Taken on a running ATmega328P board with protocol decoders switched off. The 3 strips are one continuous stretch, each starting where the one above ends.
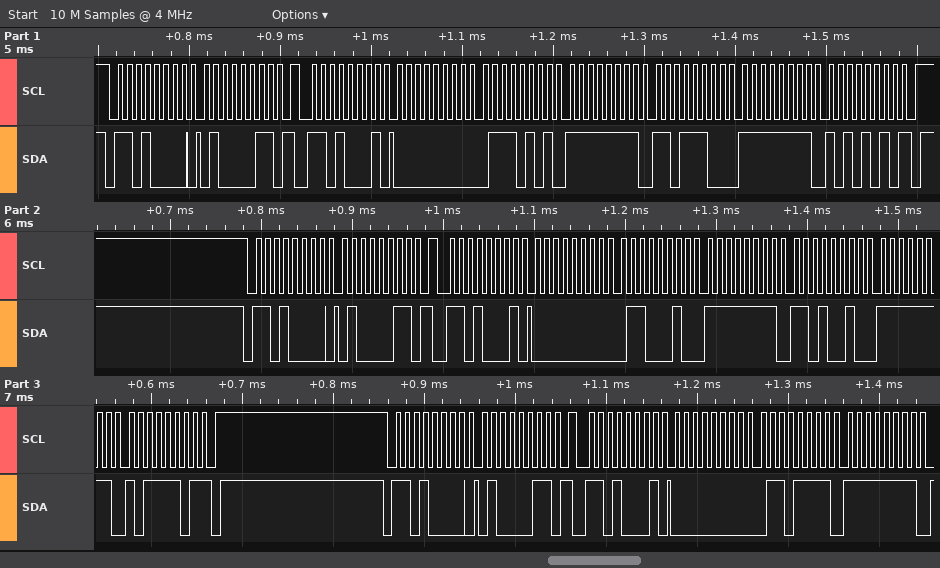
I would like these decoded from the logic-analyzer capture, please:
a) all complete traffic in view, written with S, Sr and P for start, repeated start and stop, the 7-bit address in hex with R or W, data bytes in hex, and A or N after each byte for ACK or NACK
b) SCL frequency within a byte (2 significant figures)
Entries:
S 68W A 43 A Sr 68R A 00 A 75 A FF A DC A FF A AA N P S 68W A 43 A Sr 68R A 00 A 62 A FF A D2 A FF A BD N P S 68W A 43 A Sr 68R A 00 A 6F A FF A
100 kHz
